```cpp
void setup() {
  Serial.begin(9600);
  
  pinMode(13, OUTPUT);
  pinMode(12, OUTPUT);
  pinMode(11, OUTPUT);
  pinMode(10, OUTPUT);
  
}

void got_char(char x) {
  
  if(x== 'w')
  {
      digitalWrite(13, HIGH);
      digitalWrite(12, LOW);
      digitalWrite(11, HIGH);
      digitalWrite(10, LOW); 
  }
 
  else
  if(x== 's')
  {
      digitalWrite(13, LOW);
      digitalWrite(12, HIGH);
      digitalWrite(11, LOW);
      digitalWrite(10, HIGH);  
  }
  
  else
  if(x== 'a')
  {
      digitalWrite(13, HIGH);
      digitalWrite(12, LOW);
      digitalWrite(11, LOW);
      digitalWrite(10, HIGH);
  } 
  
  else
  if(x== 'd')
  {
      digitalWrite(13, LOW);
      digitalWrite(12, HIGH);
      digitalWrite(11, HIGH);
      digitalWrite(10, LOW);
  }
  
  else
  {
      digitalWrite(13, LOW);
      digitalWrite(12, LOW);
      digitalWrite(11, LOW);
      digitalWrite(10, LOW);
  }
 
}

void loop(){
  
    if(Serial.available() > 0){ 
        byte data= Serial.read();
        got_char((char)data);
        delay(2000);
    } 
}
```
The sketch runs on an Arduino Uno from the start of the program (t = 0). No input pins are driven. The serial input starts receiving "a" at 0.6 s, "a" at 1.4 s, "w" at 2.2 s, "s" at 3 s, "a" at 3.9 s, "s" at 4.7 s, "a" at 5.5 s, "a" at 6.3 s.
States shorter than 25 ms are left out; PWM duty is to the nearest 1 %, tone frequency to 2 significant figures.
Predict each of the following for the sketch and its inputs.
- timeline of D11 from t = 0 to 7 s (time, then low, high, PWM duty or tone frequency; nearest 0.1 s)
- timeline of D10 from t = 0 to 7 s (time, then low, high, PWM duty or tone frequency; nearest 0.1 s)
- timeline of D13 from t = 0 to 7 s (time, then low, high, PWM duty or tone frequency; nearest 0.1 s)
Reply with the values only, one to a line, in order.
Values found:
0 s low; 4.6 s high; 6.6 s low
0 s low; 0.6 s high; 4.6 s low; 6.6 s high
0 s low; 0.6 s high; 6.6 s low
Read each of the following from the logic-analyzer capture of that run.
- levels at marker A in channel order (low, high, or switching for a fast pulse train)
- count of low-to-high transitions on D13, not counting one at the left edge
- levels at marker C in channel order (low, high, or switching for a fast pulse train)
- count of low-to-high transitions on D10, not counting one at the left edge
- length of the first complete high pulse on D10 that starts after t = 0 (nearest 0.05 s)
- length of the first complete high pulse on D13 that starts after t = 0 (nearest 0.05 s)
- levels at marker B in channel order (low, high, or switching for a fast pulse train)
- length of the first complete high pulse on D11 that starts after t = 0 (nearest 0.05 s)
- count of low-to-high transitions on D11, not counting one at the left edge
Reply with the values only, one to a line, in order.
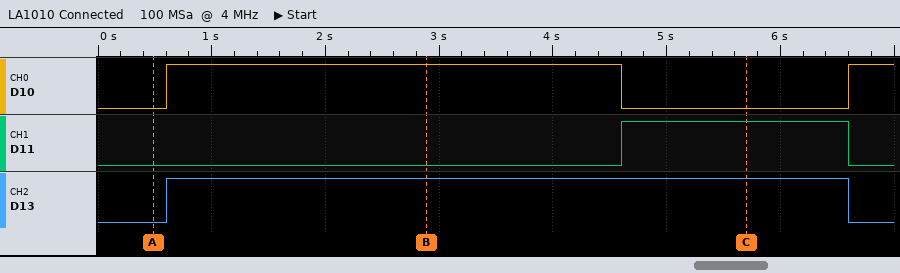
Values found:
D10 low, D11 low, D13 low
1
D10 low, D11 high, D13 high
2
4.00 s
6.00 s
D10 high, D11 low, D13 high
2.00 s
1
